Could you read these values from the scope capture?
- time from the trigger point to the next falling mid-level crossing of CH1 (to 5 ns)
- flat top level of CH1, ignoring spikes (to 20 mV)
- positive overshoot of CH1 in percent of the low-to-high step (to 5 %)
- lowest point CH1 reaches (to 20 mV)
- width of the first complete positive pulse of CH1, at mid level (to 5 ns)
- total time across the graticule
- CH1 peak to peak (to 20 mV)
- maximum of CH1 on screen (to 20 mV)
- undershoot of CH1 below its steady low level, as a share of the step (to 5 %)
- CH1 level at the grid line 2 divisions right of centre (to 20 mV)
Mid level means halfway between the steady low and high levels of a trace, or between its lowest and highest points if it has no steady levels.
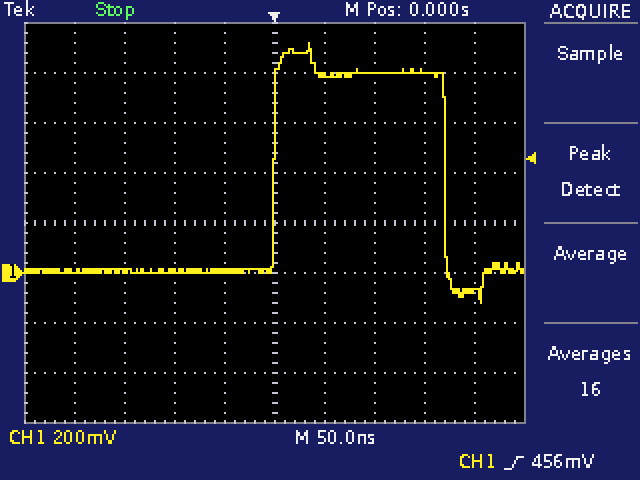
170 ns
800 mV
15 %
-120 mV
170 ns
500 ns
1.04 V
920 mV
15 %
800 mV
